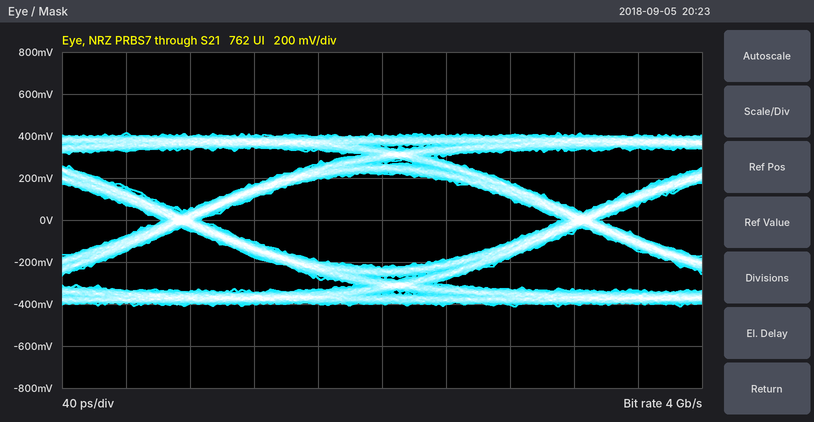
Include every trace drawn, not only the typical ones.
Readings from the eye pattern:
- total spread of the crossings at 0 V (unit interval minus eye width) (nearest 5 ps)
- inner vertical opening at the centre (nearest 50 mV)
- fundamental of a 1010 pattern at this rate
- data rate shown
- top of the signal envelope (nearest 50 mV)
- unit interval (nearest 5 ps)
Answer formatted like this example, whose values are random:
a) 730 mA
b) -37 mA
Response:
a) 25 ps
b) 450 mV
c) 2 GHz
d) 4 Gb/s
e) 400 mV
f) 250 ps
